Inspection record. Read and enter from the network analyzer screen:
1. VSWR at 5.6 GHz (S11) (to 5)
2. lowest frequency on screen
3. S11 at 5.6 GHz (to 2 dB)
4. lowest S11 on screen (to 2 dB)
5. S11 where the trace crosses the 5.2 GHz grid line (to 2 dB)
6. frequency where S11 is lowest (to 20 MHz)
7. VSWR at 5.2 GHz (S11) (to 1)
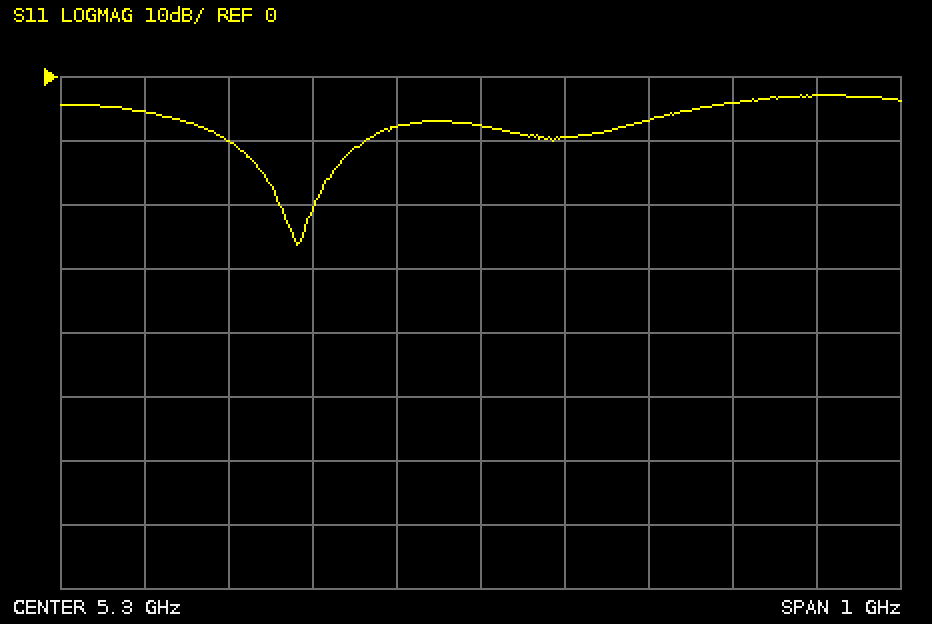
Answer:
5
4.8 GHz
-4 dB
-26 dB
-8 dB
5.08 GHz
2
